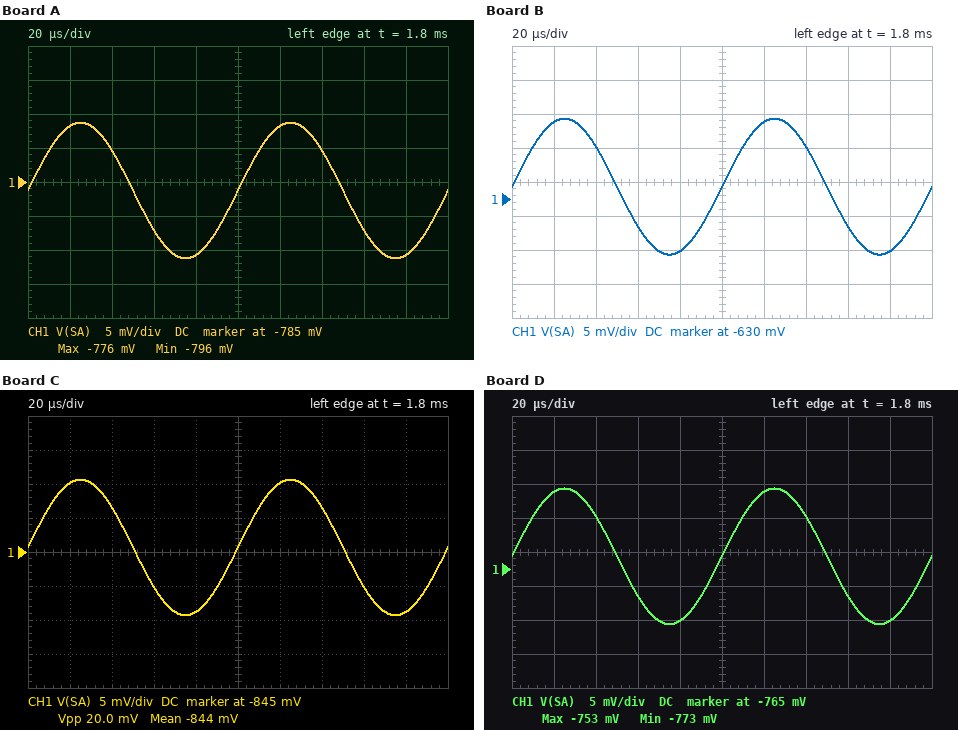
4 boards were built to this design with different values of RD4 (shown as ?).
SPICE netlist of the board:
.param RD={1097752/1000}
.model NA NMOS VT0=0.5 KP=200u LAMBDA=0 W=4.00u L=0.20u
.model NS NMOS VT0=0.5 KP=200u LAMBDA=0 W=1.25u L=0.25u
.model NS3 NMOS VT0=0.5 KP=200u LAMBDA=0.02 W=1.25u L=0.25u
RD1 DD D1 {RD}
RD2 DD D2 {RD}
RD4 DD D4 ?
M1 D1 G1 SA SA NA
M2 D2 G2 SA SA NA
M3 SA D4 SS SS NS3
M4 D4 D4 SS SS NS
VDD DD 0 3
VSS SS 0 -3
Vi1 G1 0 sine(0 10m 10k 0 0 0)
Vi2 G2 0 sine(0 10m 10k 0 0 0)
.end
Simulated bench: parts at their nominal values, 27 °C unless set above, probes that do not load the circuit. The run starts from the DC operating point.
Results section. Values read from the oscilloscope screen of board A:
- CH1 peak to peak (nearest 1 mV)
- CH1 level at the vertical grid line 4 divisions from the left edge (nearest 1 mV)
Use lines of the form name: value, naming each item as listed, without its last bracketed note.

CH1 peak to peak: 20 mV
CH1 level at the vertical grid line 4 divisions from the left edge: -796 mV
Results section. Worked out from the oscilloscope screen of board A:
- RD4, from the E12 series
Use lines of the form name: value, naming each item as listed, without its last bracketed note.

RD4, from the E12 series: 15 kΩ
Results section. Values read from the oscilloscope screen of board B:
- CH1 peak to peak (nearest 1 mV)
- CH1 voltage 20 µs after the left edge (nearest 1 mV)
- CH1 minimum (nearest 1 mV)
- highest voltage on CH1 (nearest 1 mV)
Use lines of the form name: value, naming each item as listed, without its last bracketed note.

CH1 peak to peak: 20 mV
CH1 voltage 20 µs after the left edge: -619 mV
CH1 minimum: -638 mV
highest voltage on CH1: -618 mV
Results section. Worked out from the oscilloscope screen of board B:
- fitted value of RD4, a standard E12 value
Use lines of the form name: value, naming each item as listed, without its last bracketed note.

fitted value of RD4, a standard E12 value: 82 kΩ
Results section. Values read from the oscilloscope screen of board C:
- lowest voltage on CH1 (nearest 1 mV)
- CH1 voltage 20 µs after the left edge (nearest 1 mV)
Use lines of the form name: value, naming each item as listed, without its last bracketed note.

lowest voltage on CH1: -854 mV
CH1 voltage 20 µs after the left edge: -835 mV
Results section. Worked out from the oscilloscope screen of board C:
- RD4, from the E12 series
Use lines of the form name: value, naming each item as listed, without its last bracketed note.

RD4, from the E12 series: 10 kΩ
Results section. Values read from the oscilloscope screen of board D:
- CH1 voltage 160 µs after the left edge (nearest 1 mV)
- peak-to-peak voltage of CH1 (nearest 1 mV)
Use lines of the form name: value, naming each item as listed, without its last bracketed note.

CH1 voltage 160 µs after the left edge: -769 mV
peak-to-peak voltage of CH1: 20 mV
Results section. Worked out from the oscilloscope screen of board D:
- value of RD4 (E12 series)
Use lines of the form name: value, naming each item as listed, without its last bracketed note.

value of RD4: 18 kΩ
